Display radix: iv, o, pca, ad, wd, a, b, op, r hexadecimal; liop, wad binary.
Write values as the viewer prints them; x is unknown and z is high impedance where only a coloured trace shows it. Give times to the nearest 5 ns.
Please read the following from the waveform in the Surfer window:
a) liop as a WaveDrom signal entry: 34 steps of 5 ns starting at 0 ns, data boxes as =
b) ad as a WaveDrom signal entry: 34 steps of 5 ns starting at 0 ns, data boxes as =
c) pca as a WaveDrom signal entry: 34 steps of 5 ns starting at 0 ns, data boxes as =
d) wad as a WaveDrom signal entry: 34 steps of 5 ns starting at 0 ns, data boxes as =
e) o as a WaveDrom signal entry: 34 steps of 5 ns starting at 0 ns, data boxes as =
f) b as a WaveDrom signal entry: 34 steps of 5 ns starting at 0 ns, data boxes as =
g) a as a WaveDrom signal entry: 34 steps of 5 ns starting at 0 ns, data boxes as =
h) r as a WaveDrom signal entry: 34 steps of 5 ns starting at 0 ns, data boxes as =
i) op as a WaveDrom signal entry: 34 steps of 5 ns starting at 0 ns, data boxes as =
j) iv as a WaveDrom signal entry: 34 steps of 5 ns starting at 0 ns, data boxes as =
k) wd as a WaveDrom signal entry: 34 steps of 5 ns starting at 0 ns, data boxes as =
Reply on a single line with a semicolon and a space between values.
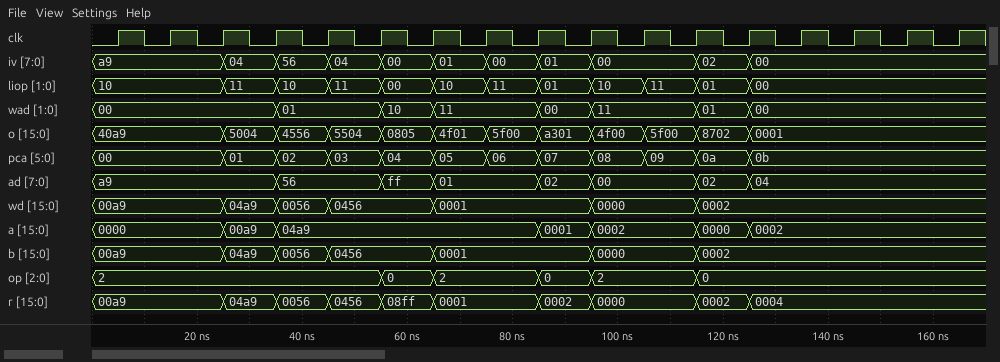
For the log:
{name: 'liop', wave: '=....=.=.=.=.=.=.=.=.=.=.=........', data: '10 11 10 11 00 10 11 01 10 11 01 00'}; {name: 'ad', wave: '=......=...=.=...=.=...=.=........', data: 'a9 56 ff 01 02 00 02 04'}; {name: 'pca', wave: '=....=.=.=.=.=.=.=.=.=.=.=........', data: '00 01 02 03 04 05 06 07 08 09 0a 0b'}; {name: 'wad', wave: '=......=...=.=...=.=...=.=........', data: '00 01 10 11 00 11 01 00'}; {name: 'o', wave: '=....=.=.=.=.=.=.=.=.=.=.=........', data: '40a9 5004 4556 5504 0805 4f01 5f00 a301 4f00 5f00 8702 0001'}; {name: 'b', wave: '=....=.=.=...=.....=...=..........', data: '00a9 04a9 0056 0456 0001 0000 0002'}; {name: 'a', wave: '=....=.=.........=.=...=.=........', data: '0000 00a9 04a9 0001 0002 0000 0002'}; {name: 'r', wave: '=....=.=.=.=.=...=.=...=.=........', data: '00a9 04a9 0056 0456 08ff 0001 0002 0000 0002 0004'}; {name: 'op', wave: '=..........=.=...=.=...=..........', data: '2 0 2 0 2 0'}; {name: 'iv', wave: '=....=.=.=.=.=.=.=.=...=.=........', data: 'a9 04 56 04 00 01 00 01 00 02 00'}; {name: 'wd', wave: '=....=.=.=...=.....=...=..........', data: '00a9 04a9 0056 0456 0001 0000 0002'}
